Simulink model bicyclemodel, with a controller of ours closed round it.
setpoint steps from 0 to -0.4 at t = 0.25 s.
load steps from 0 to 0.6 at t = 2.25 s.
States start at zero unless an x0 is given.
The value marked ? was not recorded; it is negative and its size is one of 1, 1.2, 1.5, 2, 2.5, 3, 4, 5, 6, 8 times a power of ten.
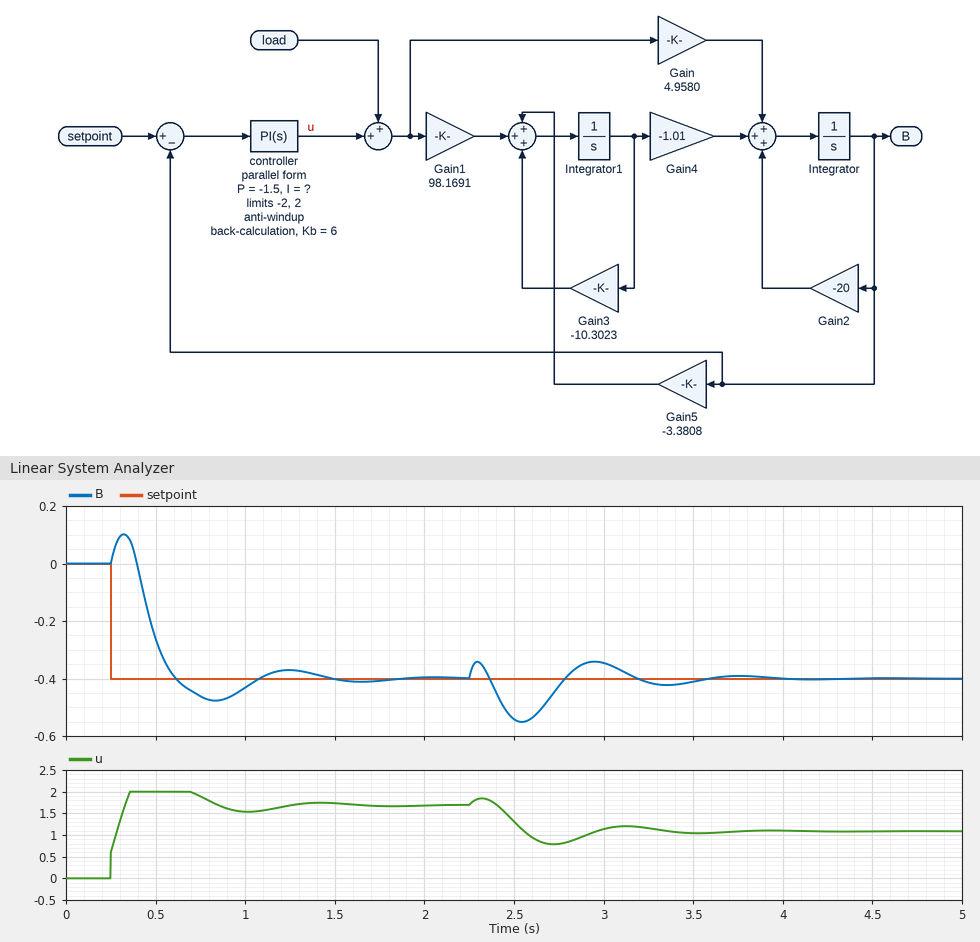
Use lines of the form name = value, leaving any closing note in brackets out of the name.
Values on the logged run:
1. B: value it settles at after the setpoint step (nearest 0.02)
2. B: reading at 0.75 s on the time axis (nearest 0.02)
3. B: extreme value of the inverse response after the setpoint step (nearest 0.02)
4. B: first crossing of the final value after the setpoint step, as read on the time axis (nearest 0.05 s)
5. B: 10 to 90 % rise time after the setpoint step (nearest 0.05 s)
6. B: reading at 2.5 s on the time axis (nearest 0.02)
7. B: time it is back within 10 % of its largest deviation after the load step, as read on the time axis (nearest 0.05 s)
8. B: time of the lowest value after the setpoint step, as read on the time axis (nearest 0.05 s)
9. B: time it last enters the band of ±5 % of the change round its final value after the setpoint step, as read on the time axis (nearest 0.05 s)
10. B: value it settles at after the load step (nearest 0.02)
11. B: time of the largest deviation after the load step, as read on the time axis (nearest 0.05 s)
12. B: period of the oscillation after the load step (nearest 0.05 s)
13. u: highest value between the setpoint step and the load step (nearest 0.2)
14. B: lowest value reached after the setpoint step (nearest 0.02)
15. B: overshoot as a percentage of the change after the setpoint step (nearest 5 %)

B: value it settles at after the setpoint step = -0.40
B: reading at 0.75 s on the time axis = -0.46
B: extreme value of the inverse response after the setpoint step = 0.10
B: first crossing of the final value after the setpoint step, as read on the time axis = 0.60 s
B: 10 to 90 % rise time after the setpoint step = 0.15 s
B: reading at 2.5 s on the time axis = -0.54
B: time it is back within 10 % of its largest deviation after the load step, as read on the time axis = 3.45 s
B: time of the lowest value after the setpoint step, as read on the time axis = 0.85 s
B: time it last enters the band of ±5 % of the change round its final value after the setpoint step, as read on the time axis = 1.35 s
B: value it settles at after the load step = -0.40
B: time of the largest deviation after the load step, as read on the time axis = 2.55 s
B: period of the oscillation after the load step = 0.80 s
u: highest value between the setpoint step and the load step = 2.0
B: lowest value reached after the setpoint step = -0.48
B: overshoot as a percentage of the change after the setpoint step = 20 %
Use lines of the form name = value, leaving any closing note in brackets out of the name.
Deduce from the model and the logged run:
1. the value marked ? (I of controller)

the value marked ? = -25
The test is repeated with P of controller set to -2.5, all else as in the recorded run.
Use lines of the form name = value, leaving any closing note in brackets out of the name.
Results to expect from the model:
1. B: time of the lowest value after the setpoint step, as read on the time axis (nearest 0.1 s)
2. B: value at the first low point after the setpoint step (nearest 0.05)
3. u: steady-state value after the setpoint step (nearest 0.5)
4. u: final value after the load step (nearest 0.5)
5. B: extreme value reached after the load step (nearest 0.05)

B: time of the lowest value after the setpoint step, as read on the time axis = 0.7 s
B: value at the first low point after the setpoint step = -0.45
u: steady-state value after the setpoint step = 1.5
u: final value after the load step = 1.0
B: extreme value reached after the load step = -0.55
